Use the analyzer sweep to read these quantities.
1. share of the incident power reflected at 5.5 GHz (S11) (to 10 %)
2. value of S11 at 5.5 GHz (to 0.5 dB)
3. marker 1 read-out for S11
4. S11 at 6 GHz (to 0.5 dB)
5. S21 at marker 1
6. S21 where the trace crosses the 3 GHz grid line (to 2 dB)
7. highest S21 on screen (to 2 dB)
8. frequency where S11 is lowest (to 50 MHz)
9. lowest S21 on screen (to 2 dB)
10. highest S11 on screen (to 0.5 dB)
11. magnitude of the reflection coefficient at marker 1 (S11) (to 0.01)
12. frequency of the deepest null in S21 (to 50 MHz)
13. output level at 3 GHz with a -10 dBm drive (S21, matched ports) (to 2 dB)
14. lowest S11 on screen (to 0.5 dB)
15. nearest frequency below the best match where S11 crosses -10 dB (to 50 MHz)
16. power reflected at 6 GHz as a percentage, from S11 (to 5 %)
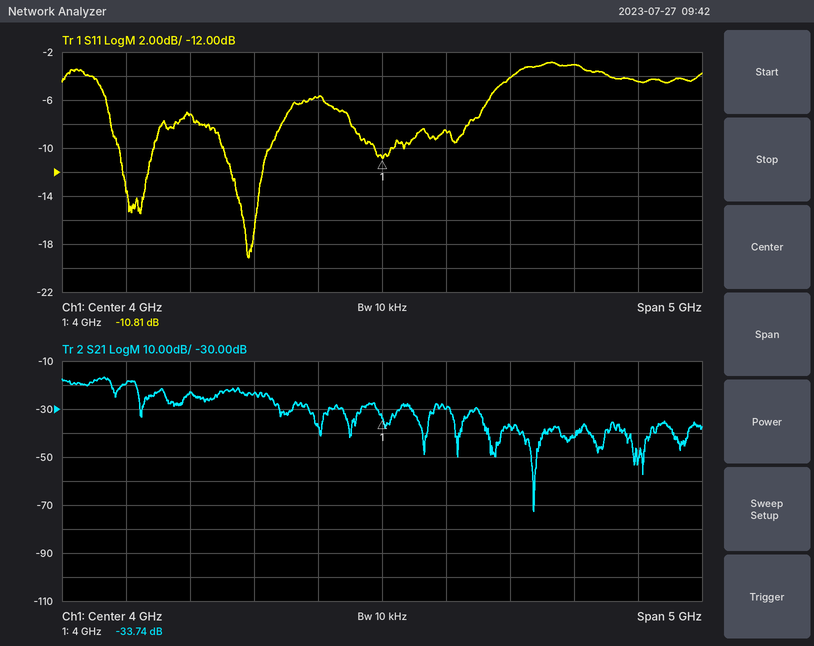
50 %
-3.0 dB
-10.81 dB
-4.5 dB
-33.74 dB
-24 dB
-16 dB
2.95 GHz
-72 dB
-3.0 dB
0.29
5.20 GHz
-34 dBm
-19.0 dB
2.75 GHz
35 %
